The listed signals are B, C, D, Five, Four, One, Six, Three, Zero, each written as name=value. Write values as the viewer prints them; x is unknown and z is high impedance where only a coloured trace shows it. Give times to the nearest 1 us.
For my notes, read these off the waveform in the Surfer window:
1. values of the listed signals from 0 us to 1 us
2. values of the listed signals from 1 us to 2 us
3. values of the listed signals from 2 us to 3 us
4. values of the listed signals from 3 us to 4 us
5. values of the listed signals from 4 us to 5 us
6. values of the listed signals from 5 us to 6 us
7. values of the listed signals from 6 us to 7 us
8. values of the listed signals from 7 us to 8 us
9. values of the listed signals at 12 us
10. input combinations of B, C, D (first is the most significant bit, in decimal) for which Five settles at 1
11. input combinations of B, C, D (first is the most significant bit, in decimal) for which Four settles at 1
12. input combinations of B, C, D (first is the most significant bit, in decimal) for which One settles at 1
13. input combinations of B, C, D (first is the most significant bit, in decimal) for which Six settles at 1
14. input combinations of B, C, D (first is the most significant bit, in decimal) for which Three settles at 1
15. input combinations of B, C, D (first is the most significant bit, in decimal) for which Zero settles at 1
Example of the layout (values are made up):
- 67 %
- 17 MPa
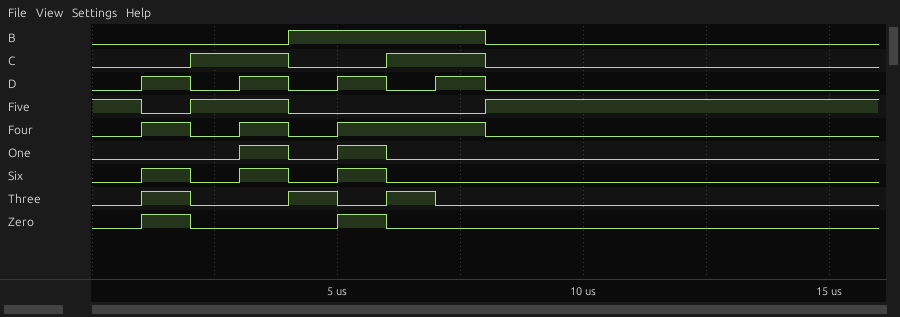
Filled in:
- B=0, C=0, D=0, Five=1, Four=0, One=0, Six=0, Three=0, Zero=0
- B=0, C=0, D=1, Five=0, Four=1, One=0, Six=1, Three=1, Zero=1
- B=0, C=1, D=0, Five=1, Four=0, One=0, Six=0, Three=0, Zero=0
- B=0, C=1, D=1, Five=1, Four=1, One=1, Six=1, Three=0, Zero=0
- B=1, C=0, D=0, Five=0, Four=0, One=0, Six=0, Three=1, Zero=0
- B=1, C=0, D=1, Five=0, Four=1, One=1, Six=1, Three=0, Zero=1
- B=1, C=1, D=0, Five=0, Four=1, One=0, Six=0, Three=1, Zero=0
- B=1, C=1, D=1, Five=0, Four=1, One=0, Six=0, Three=0, Zero=0
- B=0, C=0, D=0, Five=1, Four=0, One=0, Six=0, Three=0, Zero=0
- 0, 2, 3
- 1, 3, 5, 6, 7
- 3, 5
- 1, 3, 5
- 1, 4, 6
- 1, 5
